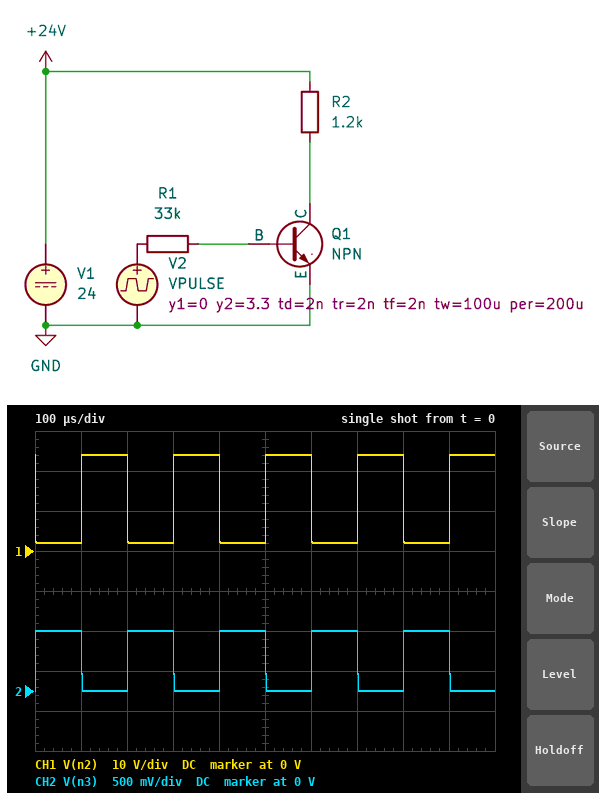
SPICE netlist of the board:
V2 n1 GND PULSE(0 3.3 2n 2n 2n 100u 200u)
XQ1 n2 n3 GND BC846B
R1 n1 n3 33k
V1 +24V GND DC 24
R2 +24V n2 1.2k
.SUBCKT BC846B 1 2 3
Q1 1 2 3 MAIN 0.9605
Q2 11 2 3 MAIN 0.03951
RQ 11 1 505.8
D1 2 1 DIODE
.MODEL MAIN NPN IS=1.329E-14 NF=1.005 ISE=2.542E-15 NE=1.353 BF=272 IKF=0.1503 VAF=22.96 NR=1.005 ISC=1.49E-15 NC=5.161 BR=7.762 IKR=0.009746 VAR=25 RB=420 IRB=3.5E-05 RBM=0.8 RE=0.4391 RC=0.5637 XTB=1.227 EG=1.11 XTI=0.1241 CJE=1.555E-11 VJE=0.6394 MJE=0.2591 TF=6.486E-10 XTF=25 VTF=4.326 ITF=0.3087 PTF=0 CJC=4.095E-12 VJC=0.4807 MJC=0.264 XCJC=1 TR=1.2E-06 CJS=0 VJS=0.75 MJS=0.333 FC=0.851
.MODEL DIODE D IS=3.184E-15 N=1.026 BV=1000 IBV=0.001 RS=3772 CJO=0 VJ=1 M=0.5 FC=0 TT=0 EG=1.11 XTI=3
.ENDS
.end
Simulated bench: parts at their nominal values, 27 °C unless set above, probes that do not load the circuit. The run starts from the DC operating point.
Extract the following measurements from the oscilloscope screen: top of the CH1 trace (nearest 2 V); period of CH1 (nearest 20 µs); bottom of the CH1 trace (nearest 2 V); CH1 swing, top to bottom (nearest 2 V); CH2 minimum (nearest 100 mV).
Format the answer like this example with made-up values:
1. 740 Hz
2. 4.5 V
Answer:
1. 24 V
2. 200 µs
3. 2 V
4. 22 V
5. 0 V
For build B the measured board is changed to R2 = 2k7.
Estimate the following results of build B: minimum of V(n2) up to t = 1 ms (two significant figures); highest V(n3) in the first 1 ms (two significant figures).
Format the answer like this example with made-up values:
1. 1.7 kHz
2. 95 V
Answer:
1. 110 mV
2. 730 mV
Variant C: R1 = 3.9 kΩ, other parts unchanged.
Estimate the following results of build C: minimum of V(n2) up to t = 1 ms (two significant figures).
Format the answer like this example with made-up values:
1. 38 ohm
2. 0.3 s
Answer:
1. 78 mV
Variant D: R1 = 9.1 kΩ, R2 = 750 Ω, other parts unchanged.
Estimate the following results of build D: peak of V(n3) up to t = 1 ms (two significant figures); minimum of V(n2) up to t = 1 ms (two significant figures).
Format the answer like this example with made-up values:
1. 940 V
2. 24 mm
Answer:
1. 800 mV
2. 150 mV
